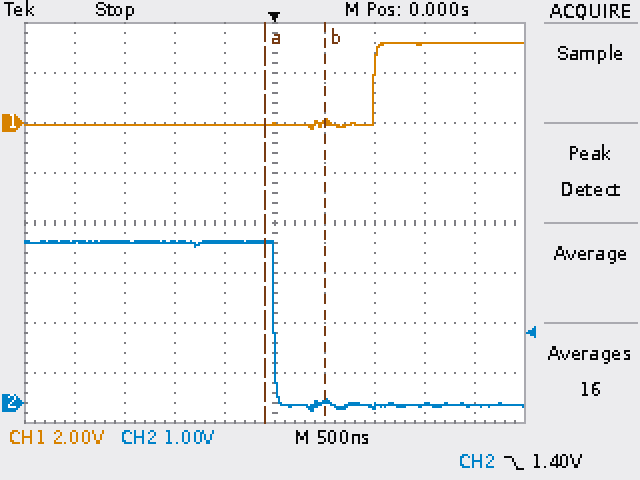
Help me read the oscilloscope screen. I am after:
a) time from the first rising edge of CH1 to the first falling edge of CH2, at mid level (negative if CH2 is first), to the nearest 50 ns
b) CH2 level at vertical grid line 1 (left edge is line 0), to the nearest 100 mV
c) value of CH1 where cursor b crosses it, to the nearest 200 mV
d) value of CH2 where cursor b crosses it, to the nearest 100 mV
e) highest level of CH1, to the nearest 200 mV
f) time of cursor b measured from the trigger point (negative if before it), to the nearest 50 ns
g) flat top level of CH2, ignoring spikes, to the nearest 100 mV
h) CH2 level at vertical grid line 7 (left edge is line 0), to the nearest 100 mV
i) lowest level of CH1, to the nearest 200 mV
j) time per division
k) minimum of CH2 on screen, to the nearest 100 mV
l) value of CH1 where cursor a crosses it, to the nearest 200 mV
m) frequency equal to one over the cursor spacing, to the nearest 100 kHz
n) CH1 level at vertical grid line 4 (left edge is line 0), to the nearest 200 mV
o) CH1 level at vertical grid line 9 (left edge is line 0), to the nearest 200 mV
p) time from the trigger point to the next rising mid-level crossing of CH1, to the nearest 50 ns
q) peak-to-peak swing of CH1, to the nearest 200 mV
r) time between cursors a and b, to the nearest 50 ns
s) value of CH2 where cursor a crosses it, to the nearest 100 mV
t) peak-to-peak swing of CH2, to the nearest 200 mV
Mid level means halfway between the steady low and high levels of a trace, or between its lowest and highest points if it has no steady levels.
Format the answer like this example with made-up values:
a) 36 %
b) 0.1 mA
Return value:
a) -1.00 µs
b) 3.2 V
c) 0.0 V
d) 0.0 V
e) 3.2 V
f) +500 ns
g) 3.2 V
h) -100 mV
i) -200 mV
j) 500 ns
k) -200 mV
l) 0.0 V
m) 1.7 MHz
n) 0.0 V
o) 3.2 V
p) 1.00 µs
q) 3.4 V
r) 600 ns
s) 3.2 V
t) 3.4 V
